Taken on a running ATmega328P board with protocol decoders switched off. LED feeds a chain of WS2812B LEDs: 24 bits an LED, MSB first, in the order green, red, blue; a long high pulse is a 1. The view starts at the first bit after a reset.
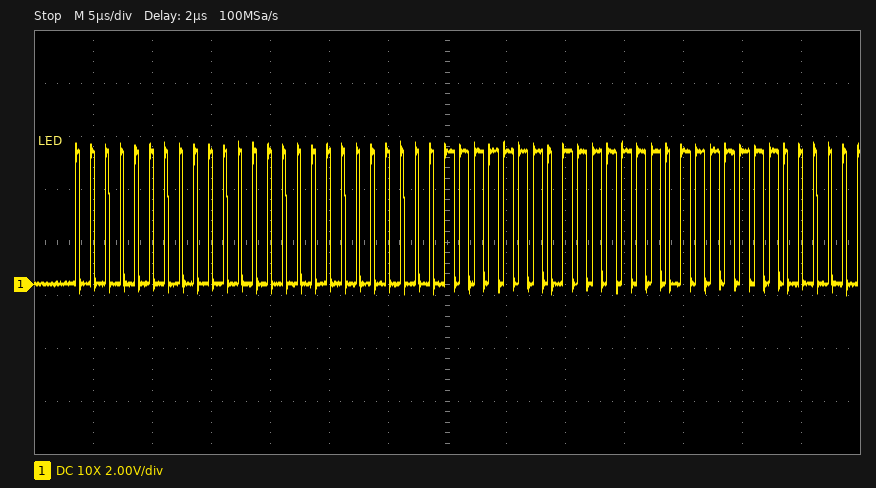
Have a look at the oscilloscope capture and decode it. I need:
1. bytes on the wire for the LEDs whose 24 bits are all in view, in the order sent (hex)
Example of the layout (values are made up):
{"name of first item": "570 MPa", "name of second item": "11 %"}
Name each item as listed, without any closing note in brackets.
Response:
{"bytes on the wire for the LEDs whose 24 bits are all in view, in the order sent": "00 00 00 7F 7F 7F"}
